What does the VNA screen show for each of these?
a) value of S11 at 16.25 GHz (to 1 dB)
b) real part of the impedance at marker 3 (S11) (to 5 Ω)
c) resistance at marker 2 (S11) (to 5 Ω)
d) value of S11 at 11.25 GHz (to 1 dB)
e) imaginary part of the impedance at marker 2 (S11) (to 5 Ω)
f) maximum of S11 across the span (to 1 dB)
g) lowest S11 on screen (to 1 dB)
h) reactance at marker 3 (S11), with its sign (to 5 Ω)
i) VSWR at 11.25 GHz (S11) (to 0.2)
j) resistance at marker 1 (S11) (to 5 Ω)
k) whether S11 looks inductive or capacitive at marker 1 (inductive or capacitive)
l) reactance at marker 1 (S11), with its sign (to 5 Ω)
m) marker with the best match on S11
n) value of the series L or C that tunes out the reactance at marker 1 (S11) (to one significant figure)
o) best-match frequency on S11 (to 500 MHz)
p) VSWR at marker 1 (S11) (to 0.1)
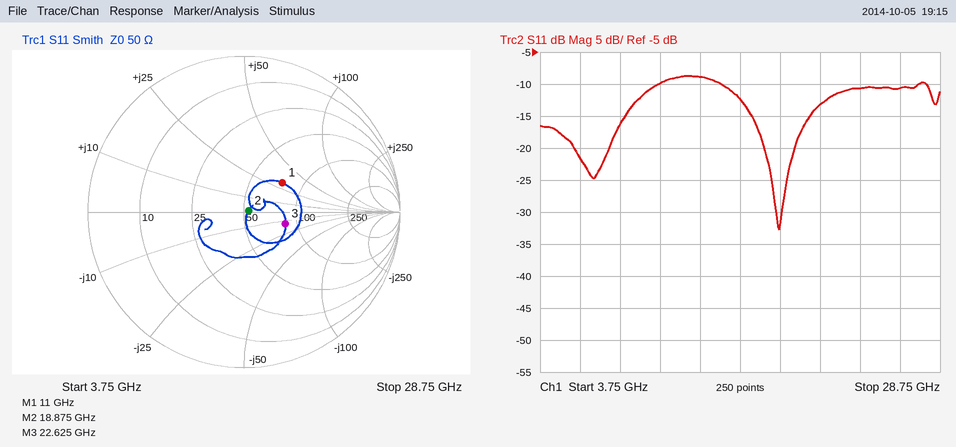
-12 dB
85 Ω
55 Ω
-10 dB
0 Ω
-9 dB
-33 dB
-15 Ω
2.0
75 Ω
inductive
+30 Ω
marker 2
500 fF
18.5 GHz
1.9
